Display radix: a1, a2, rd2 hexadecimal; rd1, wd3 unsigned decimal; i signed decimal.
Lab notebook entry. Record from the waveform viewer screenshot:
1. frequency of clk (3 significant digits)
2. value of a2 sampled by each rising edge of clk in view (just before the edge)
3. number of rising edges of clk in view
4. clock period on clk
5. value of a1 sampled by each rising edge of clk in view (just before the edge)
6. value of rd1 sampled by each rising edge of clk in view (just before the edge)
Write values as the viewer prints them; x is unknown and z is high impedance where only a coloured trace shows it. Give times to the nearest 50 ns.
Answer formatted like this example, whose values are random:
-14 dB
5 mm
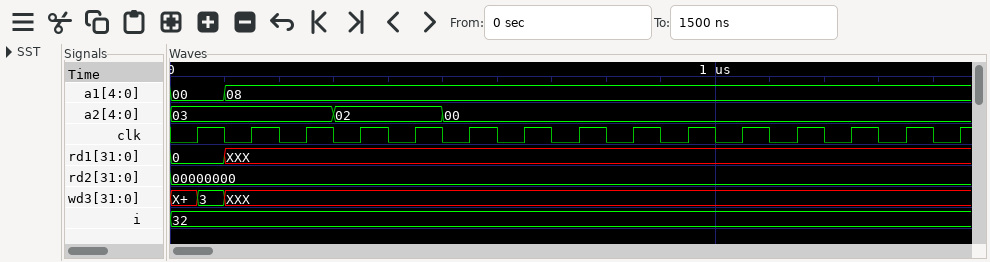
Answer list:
10.0 MHz
03, 03, 03, 02, 02, 00, 00, 00, 00, 00, 00, 00, 00, 00, 00
15
100 ns
00, 08, 08, 08, 08, 08, 08, 08, 08, 08, 08, 08, 08, 08, 08
0, XXX, XXX, XXX, XXX, XXX, XXX, XXX, XXX, XXX, XXX, XXX, XXX, XXX, XXX
